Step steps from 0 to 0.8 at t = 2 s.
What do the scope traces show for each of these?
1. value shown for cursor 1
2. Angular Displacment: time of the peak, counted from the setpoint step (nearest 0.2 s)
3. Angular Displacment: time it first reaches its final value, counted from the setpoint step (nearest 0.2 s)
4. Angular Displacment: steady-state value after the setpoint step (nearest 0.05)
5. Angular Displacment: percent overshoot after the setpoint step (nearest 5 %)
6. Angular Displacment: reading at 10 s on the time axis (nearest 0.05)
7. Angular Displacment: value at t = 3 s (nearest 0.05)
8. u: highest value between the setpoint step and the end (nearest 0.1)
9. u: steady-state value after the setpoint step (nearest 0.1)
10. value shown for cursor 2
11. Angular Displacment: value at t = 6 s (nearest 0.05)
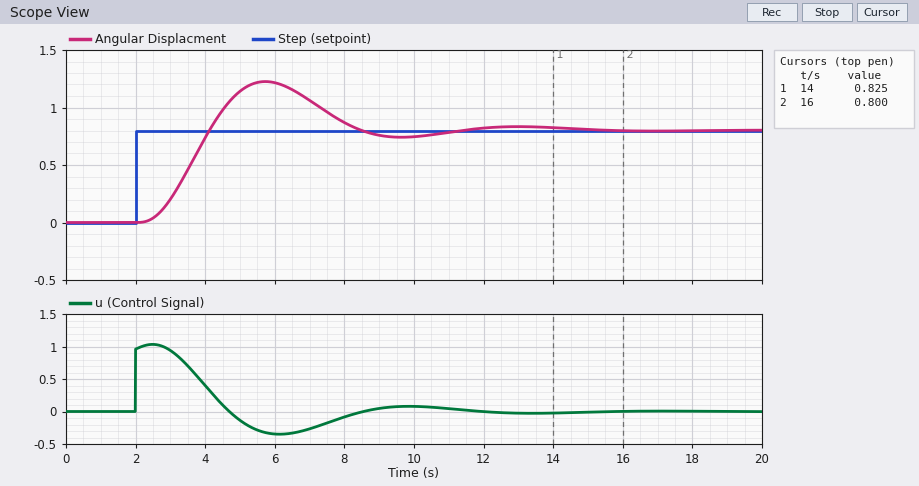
0.825
3.8 s
2.2 s
0.80
55 %
0.75
0.20
1.0
0.0
0.800
1.20
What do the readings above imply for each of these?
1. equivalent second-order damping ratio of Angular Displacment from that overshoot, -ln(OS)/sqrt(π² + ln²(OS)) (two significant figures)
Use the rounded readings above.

0.19
